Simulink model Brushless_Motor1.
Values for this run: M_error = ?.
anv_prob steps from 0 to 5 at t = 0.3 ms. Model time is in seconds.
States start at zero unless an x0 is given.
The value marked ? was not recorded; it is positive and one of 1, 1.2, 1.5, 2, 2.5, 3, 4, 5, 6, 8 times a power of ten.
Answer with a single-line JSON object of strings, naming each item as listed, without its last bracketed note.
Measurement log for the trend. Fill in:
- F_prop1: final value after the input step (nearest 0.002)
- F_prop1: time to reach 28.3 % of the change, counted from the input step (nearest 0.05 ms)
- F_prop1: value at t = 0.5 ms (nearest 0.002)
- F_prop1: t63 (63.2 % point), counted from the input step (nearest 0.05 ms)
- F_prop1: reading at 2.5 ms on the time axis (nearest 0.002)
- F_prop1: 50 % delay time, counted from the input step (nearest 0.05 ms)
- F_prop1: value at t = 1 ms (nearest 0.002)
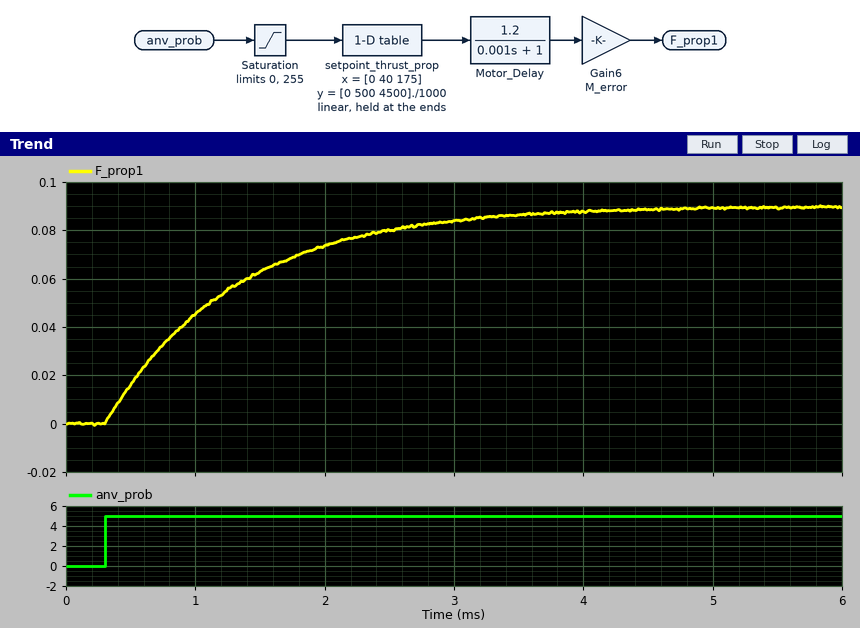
{"F_prop1: final value after the input step": "0.090", "F_prop1: time to reach 28.3 % of the change, counted from the input step": "0.35 ms", "F_prop1: value at t = 0.5 ms": "0.016", "F_prop1: t63 (63.2 % point), counted from the input step": "1.00 ms", "F_prop1: reading at 2.5 ms on the time axis": "0.080", "F_prop1: 50 % delay time, counted from the input step": "0.70 ms", "F_prop1: value at t = 1 ms": "0.046"}
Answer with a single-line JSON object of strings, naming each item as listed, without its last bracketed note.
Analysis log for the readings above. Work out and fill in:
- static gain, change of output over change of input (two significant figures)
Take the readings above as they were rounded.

{"static gain, change of output over change of input": "0.018"}
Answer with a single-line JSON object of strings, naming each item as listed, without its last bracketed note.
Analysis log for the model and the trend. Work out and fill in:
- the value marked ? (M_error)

{"the value marked ?": "1.2"}
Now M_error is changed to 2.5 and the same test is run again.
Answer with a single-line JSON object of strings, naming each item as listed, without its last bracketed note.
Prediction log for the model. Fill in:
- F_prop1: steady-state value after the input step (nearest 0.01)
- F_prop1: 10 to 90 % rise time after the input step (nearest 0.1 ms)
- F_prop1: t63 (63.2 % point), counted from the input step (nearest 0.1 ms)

{"F_prop1: steady-state value after the input step": "0.19", "F_prop1: 10 to 90 % rise time after the input step": "2.2 ms", "F_prop1: t63 (63.2 % point), counted from the input step": "1.0 ms"}
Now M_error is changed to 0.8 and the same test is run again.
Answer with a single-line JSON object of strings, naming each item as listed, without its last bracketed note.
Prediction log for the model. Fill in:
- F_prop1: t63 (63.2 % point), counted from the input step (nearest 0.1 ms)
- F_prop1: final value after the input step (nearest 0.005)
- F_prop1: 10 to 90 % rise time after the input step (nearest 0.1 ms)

{"F_prop1: t63 (63.2 % point), counted from the input step": "1.0 ms", "F_prop1: final value after the input step": "0.060", "F_prop1: 10 to 90 % rise time after the input step": "2.2 ms"}
